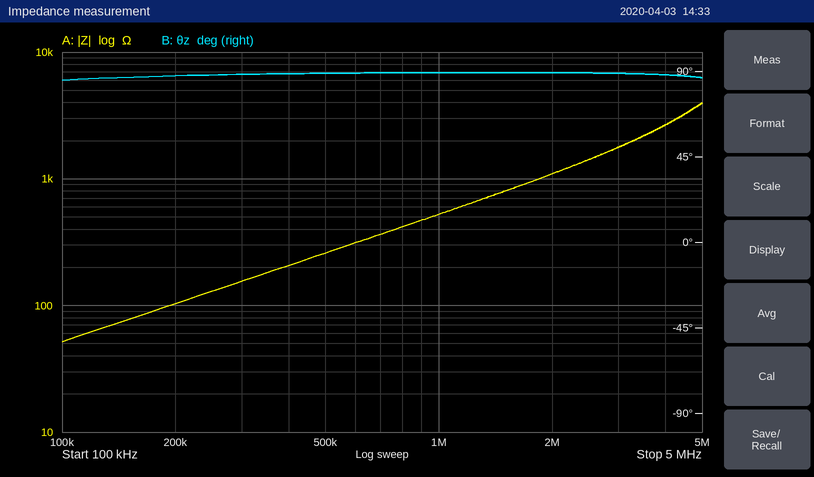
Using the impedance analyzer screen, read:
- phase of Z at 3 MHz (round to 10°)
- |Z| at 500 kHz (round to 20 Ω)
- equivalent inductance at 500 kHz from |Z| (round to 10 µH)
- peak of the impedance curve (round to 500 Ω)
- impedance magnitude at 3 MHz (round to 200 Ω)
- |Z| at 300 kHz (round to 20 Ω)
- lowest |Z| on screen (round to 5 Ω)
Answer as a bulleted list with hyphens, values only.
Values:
- 90°
- 260 Ω
- 80 µH
- 4.0 kΩ
- 1.8 kΩ
- 160 Ω
- 50 Ω
